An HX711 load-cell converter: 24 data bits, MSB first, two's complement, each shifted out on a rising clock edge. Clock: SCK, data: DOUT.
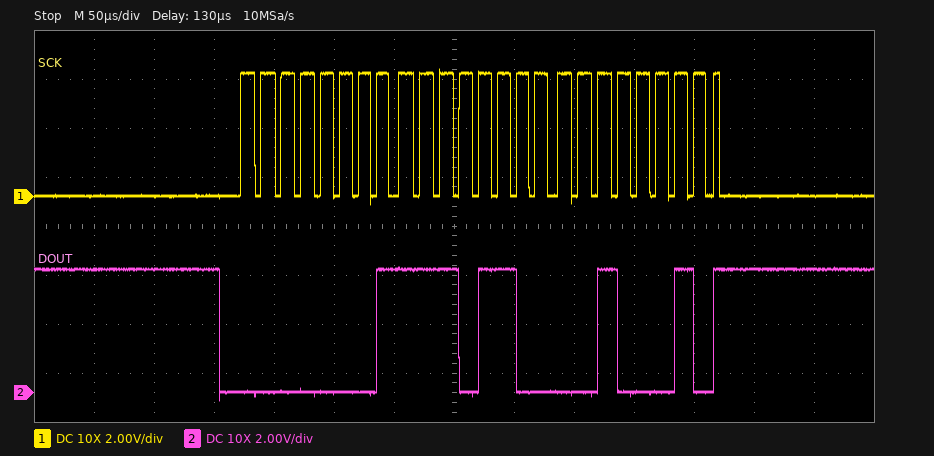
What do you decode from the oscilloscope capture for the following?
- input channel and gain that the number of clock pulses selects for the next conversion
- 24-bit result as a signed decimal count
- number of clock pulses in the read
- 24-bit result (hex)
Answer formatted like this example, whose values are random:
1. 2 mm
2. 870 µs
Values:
1. channel A, gain 128
2. 125986
3. 25
4. 0x01EC22
